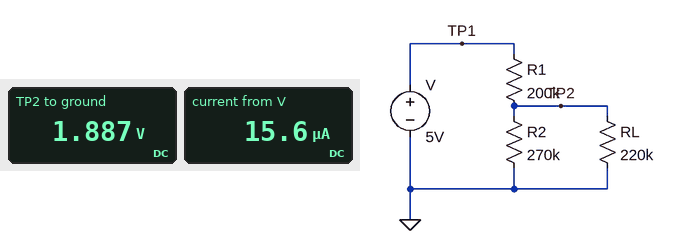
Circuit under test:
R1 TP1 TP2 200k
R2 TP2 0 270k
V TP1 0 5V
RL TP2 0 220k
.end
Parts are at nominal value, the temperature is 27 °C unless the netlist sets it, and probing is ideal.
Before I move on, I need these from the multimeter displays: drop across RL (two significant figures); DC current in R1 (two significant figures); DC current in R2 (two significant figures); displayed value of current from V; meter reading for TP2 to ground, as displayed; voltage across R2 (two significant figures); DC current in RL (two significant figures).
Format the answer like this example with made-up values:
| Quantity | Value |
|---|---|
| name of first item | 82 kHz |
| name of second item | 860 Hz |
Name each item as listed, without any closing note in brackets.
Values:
| Quantity | Value |
|---|---|
| drop across RL | 1.9 V |
| DC current in R1 | 16 µA |
| DC current in R2 | 7.0 µA |
| displayed value of current from V | 15.6 µA |
| meter reading for TP2 to ground, as displayed | 1.887 V |
| voltage across R2 | 1.9 V |
| DC current in RL | 8.6 µA |
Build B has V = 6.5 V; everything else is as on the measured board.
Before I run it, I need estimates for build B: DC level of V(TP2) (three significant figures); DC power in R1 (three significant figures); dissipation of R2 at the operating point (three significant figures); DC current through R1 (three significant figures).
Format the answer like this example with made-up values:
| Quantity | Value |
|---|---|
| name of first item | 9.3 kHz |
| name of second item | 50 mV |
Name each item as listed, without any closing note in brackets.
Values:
| Quantity | Value |
|---|---|
| DC level of V(TP2) | 2.45 V |
| DC power in R1 | 81.9 µW |
| dissipation of R2 at the operating point | 22.3 µW |
| DC current through R1 | 20.2 µA |
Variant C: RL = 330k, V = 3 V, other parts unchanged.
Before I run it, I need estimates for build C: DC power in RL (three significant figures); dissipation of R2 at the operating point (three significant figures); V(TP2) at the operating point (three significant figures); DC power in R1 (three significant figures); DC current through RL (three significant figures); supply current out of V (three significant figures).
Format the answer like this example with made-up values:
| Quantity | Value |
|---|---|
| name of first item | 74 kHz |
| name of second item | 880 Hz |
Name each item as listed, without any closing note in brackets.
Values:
| Quantity | Value |
|---|---|
| DC power in RL | 4.95 µW |
| dissipation of R2 at the operating point | 6.05 µW |
| V(TP2) at the operating point | 1.28 V |
| DC power in R1 | 14.8 µW |
| DC current through RL | 3.87 µA |
| supply current out of V | 8.61 µA |
